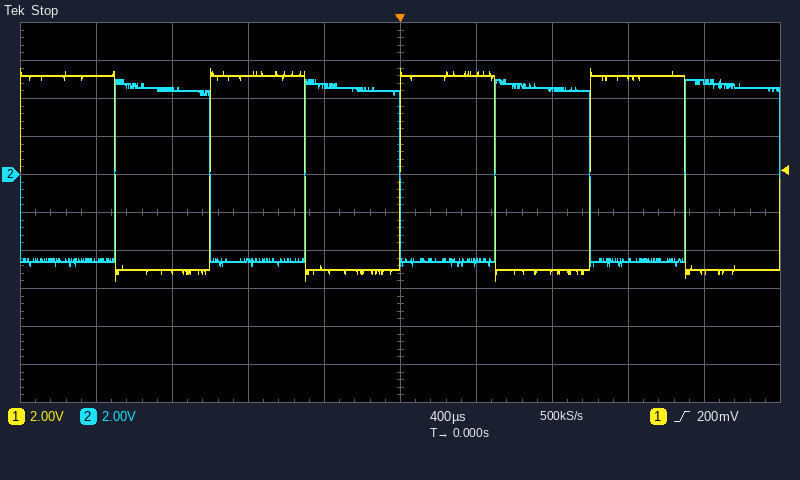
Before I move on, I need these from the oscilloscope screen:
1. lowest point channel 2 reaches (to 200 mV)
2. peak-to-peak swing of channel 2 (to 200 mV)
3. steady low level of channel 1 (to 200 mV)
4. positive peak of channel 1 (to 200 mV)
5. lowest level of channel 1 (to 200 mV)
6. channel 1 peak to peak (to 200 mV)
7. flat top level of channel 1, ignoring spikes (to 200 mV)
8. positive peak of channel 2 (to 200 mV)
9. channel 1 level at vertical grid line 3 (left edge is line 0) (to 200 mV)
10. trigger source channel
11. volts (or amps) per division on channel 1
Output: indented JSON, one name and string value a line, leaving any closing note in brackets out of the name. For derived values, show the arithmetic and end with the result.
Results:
{
  "lowest point channel 2 reaches": "-4.8 V",
  "peak-to-peak swing of channel 2": "5.0 V − (-4.8 V) = 9.8 V",
  "steady low level of channel 1": "-5.0 V",
  "positive peak of channel 1": "5.6 V",
  "lowest level of channel 1": "-5.6 V",
  "channel 1 peak to peak": "5.6 V − (-5.6 V) = 11.2 V",
  "flat top level of channel 1, ignoring spikes": "5.2 V",
  "positive peak of channel 2": "5.0 V",
  "channel 1 level at vertical grid line 3 (left edge is line 0)": "5.2 V",
  "trigger source channel": "channel 1",
  "volts (or amps) per division on channel 1": "2 V"
}
